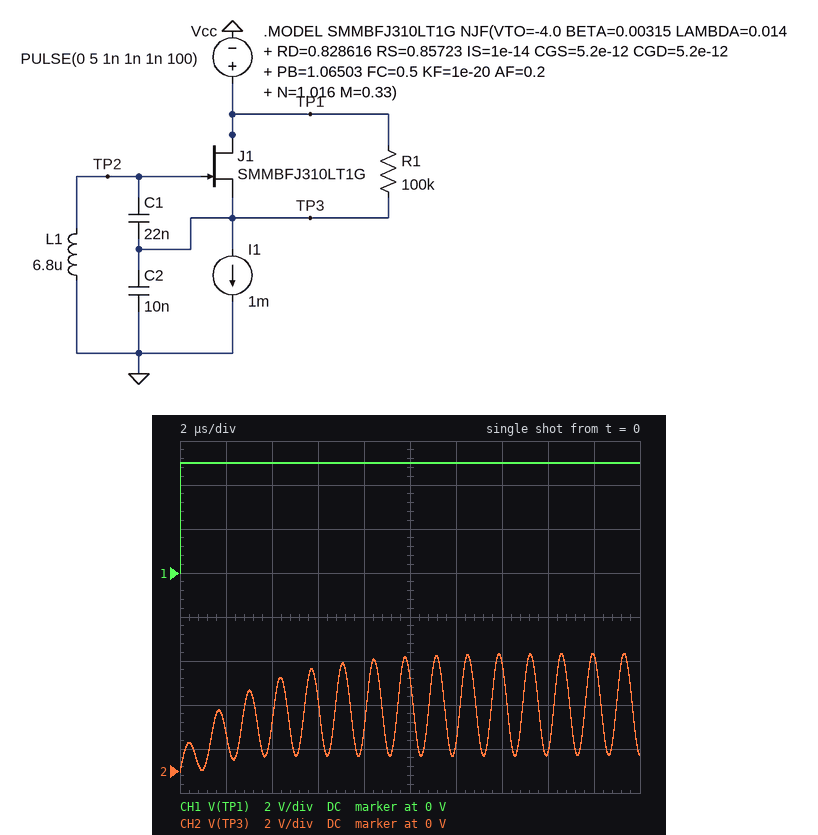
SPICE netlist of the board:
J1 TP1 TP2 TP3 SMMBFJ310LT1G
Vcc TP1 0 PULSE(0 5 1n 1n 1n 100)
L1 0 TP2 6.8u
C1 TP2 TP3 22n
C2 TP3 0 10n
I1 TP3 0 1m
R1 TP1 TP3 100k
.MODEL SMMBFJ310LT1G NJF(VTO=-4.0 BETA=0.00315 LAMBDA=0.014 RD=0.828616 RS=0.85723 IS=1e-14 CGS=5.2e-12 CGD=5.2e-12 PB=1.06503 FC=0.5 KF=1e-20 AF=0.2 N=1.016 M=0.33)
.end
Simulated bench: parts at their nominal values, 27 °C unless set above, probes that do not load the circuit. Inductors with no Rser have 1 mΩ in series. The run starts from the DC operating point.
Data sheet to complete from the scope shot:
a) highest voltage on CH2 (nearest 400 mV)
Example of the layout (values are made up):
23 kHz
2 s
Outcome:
5.2 V
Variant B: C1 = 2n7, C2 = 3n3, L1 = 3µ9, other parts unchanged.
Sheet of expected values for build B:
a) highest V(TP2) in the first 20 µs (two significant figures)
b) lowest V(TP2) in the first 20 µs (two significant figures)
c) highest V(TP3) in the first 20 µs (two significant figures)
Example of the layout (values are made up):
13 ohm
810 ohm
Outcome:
4.5 V
-4.5 V
5.3 V
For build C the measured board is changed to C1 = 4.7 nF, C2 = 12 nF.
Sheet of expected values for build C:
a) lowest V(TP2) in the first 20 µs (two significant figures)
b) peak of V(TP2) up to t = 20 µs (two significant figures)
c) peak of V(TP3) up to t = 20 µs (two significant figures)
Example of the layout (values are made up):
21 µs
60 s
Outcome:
-3.9 V
3.9 V
5.0 V
